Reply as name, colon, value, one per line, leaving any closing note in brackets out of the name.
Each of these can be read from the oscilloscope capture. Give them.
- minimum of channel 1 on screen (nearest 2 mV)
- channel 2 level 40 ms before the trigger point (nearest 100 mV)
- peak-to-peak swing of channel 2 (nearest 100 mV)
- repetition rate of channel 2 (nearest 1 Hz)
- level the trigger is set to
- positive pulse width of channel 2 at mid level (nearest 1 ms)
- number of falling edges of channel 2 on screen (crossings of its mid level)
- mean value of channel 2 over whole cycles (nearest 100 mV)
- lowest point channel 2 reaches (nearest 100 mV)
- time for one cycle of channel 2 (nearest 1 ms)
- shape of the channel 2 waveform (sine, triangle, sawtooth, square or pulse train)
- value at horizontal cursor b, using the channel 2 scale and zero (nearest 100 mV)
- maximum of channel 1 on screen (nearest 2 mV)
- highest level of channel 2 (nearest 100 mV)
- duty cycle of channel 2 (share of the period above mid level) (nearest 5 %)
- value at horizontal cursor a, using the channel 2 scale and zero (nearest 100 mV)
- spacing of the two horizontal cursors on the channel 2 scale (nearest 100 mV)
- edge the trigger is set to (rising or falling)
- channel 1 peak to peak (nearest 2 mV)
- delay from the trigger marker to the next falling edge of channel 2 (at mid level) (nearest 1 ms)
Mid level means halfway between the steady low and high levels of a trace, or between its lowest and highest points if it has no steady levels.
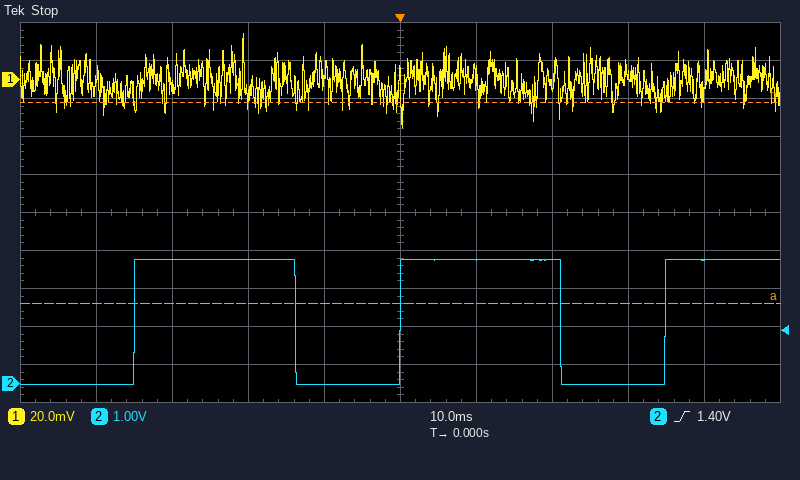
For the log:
minimum of channel 1 on screen: -26 mV
channel 2 level 40 ms before the trigger point: 0.0 V
peak-to-peak swing of channel 2: 3.3 V
repetition rate of channel 2: 29 Hz
level the trigger is set to: 1.40 V
positive pulse width of channel 2 at mid level: 21 ms
number of falling edges of channel 2 on screen: 2
mean value of channel 2 over whole cycles: 2.0 V
lowest point channel 2 reaches: 0.0 V
time for one cycle of channel 2: 35 ms
shape of the channel 2 waveform: pulse train
value at horizontal cursor b, using the channel 2 scale and zero: 7.4 V
maximum of channel 1 on screen: 24 mV
highest level of channel 2: 3.3 V
duty cycle of channel 2 (share of the period above mid level): 60 %
value at horizontal cursor a, using the channel 2 scale and zero: 2.1 V
spacing of the two horizontal cursors on the channel 2 scale: 5.3 V
edge the trigger is set to: rising
channel 1 peak to peak: 50 mV
delay from the trigger marker to the next falling edge of channel 2 (at mid level): 21 ms
